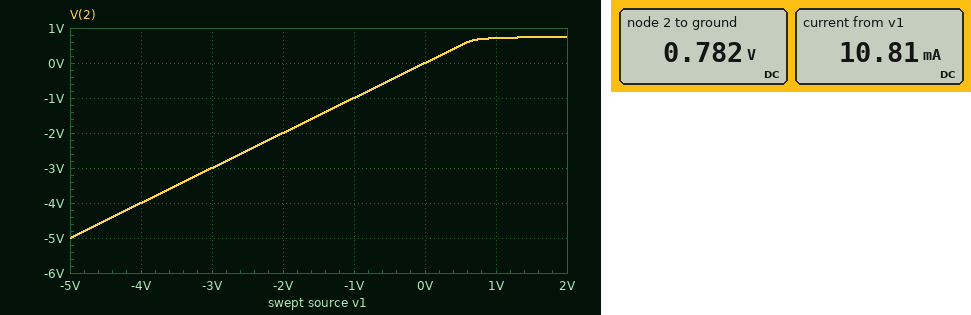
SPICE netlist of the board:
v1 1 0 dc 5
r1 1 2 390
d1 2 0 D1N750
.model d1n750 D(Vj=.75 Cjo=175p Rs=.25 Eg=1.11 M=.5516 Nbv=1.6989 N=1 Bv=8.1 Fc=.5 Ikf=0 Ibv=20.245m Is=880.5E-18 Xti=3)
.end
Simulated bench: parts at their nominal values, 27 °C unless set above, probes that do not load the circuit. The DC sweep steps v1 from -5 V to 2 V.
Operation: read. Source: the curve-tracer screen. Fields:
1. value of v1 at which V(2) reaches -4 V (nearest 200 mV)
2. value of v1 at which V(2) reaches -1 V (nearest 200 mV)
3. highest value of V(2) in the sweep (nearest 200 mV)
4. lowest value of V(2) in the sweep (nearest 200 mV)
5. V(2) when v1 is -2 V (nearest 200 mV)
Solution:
-4.0 V
-1.0 V
800 mV
-5.0 V
-2.0 V
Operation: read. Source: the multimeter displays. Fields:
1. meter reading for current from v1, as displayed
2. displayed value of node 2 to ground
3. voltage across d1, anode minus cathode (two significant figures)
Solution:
10.81 mA
0.782 V
780 mV
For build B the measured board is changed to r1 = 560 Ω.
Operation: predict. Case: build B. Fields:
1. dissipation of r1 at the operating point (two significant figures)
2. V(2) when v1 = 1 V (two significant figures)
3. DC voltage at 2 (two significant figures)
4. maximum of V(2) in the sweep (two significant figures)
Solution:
32 mW
700 mV
770 mV
740 mV
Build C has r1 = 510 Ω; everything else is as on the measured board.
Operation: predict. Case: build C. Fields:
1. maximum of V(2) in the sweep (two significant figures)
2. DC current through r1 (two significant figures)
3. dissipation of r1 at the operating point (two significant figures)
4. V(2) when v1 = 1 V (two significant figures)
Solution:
740 mV
8.3 mA
35 mW
700 mV
